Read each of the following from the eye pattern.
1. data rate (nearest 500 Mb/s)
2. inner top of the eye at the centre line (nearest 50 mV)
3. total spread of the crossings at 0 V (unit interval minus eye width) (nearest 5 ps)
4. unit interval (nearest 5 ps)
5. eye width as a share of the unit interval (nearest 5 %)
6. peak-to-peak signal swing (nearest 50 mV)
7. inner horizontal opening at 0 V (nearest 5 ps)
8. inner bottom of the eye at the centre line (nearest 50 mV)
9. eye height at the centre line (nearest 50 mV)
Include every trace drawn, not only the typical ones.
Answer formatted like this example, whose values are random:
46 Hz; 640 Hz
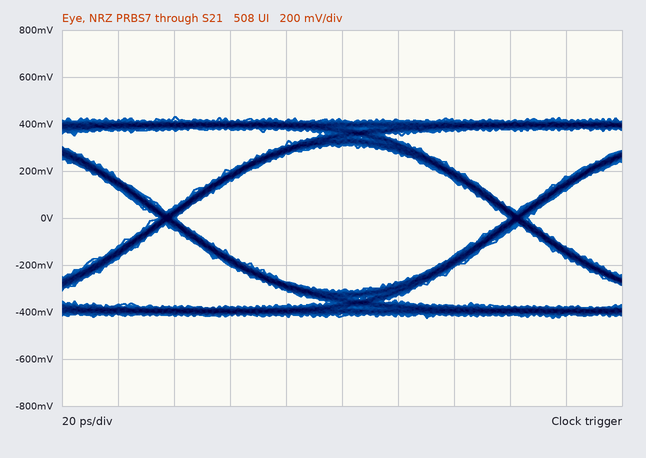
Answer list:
8.0 Gb/s; 300 mV; 5 ps; 125 ps; 95 %; 850 mV; 120 ps; -300 mV; 600 mV
